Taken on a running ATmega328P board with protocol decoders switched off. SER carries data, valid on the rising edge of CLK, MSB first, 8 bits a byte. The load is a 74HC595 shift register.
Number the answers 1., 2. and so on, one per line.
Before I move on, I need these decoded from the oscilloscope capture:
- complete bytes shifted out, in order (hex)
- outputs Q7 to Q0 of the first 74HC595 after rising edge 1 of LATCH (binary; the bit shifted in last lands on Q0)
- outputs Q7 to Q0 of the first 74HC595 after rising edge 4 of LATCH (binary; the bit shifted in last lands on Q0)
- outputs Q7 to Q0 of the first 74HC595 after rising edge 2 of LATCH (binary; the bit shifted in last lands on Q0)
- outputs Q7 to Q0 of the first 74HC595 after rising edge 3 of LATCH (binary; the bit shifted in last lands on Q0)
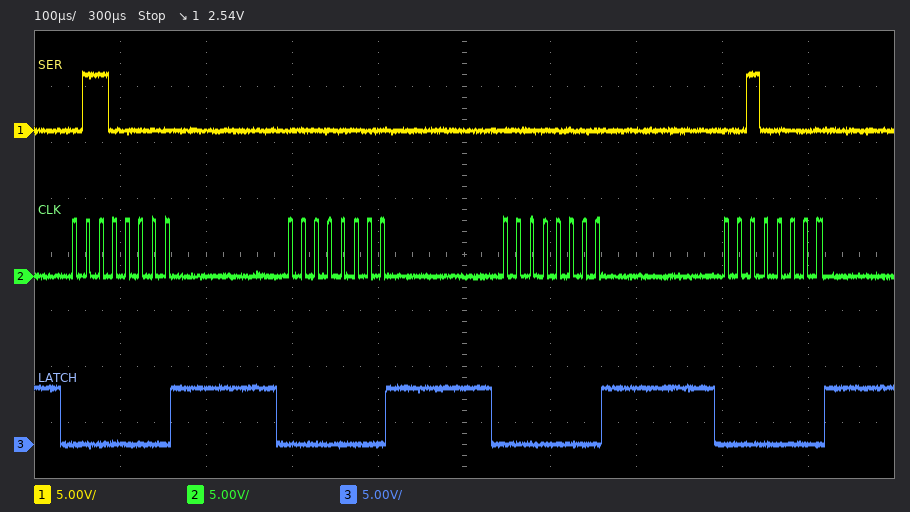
1. 60 00 00 20
2. 01100000
3. 00100000
4. 00000000
5. 00000000
